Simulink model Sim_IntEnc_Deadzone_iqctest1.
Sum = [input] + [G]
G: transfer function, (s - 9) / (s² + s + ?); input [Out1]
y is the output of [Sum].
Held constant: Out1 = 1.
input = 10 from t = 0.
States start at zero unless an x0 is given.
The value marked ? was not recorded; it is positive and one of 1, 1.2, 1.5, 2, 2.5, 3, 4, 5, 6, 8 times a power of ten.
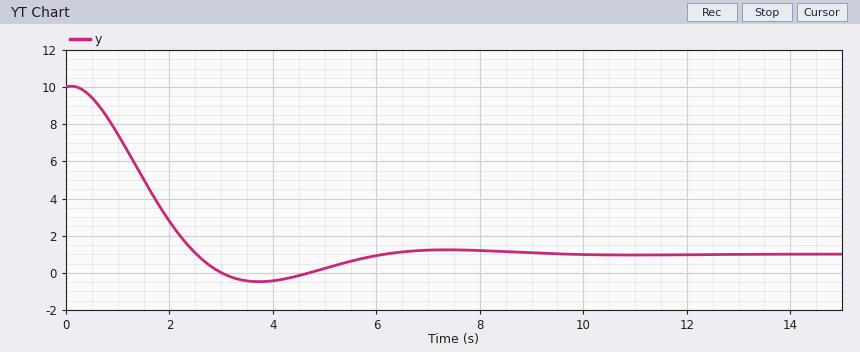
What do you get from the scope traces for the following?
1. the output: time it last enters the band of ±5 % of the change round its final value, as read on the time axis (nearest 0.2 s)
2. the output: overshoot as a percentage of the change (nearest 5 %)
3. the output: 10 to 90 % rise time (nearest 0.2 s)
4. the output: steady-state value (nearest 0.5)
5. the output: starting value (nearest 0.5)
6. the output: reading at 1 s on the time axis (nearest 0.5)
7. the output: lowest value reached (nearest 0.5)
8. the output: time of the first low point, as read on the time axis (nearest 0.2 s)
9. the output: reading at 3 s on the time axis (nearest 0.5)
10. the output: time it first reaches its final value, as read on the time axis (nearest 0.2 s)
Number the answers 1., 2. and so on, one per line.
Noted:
1. 5.4 s
2. 15 %
3. 1.6 s
4. 1.0
5. 10.0
6. 7.5
7. -0.5
8. 3.8 s
9. 0.0
10. 2.6 s
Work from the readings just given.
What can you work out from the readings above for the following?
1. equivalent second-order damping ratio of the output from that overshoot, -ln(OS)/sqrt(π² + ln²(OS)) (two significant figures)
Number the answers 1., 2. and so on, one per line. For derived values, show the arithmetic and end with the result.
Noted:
1. ln(0.15) = -1.897; 1.897 / sqrt(9.870 + 3.599) = 0.52
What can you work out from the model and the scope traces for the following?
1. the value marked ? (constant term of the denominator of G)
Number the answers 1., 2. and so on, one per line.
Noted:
1. 1
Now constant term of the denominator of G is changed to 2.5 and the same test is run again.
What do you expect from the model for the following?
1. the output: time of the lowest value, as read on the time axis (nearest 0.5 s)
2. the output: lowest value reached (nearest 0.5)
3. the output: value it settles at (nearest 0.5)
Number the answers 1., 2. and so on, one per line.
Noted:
1. 2.0 s
2. 5.0
3. 6.5
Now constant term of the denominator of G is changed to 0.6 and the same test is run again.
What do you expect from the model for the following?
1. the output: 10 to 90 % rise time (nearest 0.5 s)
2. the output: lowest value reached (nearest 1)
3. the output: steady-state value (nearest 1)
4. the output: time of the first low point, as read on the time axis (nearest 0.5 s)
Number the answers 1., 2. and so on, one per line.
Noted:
1. 2.5 s
2. -6
3. -5
4. 5.5 s
